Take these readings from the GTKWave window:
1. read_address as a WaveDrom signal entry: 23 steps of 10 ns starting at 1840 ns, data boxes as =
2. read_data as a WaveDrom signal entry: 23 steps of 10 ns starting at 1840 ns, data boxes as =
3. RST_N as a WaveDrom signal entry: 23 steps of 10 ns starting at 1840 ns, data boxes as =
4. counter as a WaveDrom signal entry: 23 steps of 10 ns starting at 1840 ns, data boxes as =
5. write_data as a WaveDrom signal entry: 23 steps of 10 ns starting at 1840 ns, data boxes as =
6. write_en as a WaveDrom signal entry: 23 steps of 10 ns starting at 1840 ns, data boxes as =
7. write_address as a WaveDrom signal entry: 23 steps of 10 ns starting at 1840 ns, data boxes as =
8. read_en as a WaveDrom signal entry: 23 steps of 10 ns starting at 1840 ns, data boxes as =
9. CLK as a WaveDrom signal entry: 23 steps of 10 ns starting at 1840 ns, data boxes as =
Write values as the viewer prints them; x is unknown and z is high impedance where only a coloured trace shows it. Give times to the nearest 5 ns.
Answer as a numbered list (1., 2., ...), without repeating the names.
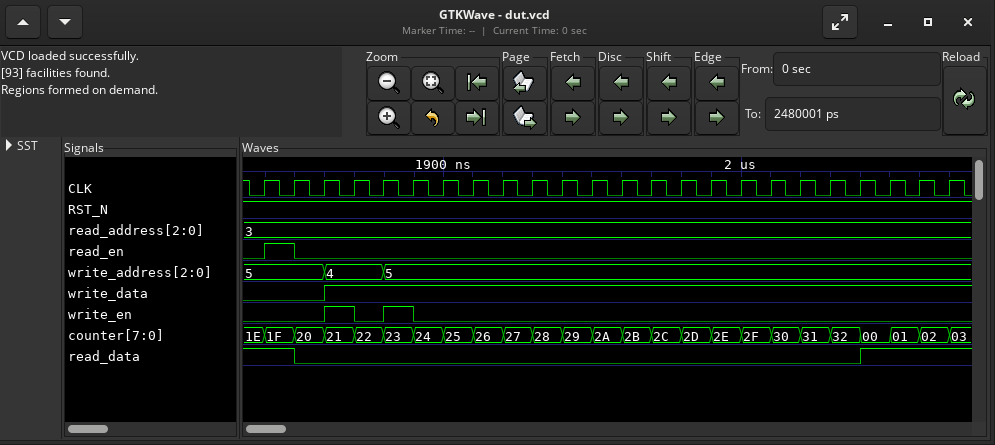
1. {name: 'read_address', wave: '=......................', data: '3'}
2. {name: 'read_data', wave: '10..................1..'}
3. {name: 'RST_N', wave: '1......................'}
4. {name: 'counter', wave: '=======================', data: '1F 20 21 22 23 24 25 26 27 28 29 2A 2B 2C 2D 2E 2F 30 31 32 00 01 02'}
5. {name: 'write_data', wave: '0.1....................'}
6. {name: 'write_en', wave: '0.1010.................'}
7. {name: 'write_address', wave: '=.=.=..................', data: '5 4 5'}
8. {name: 'read_en', wave: '10.....................'}
9. {name: 'CLK', wave: 'p......................'}
